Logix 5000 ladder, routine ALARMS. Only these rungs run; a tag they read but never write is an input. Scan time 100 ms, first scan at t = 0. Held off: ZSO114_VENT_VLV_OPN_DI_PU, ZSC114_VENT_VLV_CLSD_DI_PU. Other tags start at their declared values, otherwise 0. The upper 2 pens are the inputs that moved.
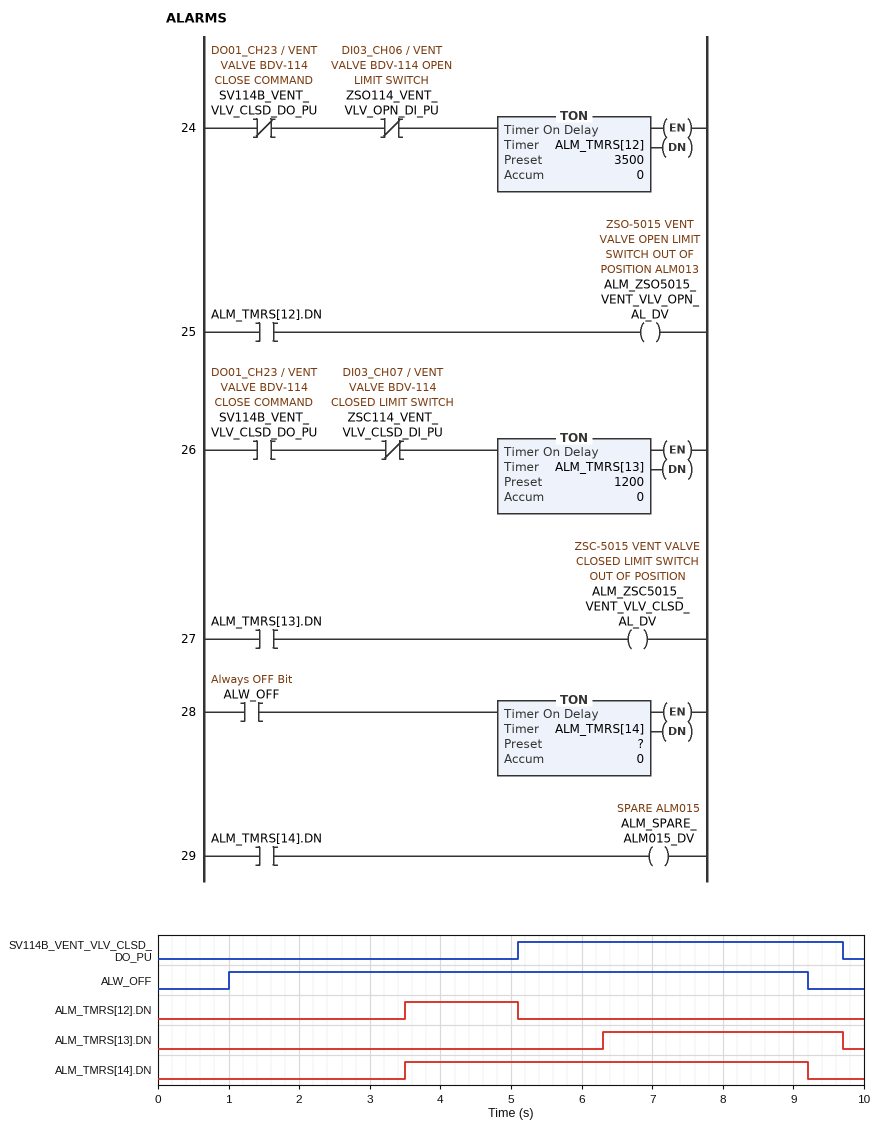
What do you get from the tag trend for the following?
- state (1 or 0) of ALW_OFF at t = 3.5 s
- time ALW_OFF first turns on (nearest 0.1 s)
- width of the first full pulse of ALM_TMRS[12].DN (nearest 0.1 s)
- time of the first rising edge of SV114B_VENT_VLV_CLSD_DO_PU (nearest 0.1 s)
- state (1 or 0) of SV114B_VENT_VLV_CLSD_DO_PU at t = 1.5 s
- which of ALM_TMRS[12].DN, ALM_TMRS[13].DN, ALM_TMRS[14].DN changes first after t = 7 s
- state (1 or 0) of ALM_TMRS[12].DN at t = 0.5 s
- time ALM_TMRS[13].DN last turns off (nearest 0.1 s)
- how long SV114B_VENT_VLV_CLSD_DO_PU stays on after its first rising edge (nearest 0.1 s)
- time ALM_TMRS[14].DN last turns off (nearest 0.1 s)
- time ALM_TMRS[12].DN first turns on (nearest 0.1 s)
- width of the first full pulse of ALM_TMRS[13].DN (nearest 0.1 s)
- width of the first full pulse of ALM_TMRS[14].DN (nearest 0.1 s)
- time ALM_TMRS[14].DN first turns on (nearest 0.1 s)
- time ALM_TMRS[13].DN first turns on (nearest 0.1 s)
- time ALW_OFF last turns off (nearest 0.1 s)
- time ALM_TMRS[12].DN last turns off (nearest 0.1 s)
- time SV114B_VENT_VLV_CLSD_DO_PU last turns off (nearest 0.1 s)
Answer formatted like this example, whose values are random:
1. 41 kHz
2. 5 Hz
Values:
1. 1
2. 1.0 s
3. 1.6 s
4. 5.1 s
5. 0
6. ALM_TMRS[14].DN
7. 0
8. 9.7 s
9. 4.6 s
10. 9.2 s
11. 3.5 s
12. 3.4 s
13. 5.7 s
14. 3.5 s
15. 6.3 s
16. 9.2 s
17. 5.1 s
18. 9.7 s
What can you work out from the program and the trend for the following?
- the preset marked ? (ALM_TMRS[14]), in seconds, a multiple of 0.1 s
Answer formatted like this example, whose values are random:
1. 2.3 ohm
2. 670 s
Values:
1. 2.5 s
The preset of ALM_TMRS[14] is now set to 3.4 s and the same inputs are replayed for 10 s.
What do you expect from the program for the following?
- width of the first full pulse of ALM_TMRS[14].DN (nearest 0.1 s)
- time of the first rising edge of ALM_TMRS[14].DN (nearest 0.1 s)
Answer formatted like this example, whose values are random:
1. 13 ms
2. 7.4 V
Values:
1. 4.8 s
2. 4.4 s
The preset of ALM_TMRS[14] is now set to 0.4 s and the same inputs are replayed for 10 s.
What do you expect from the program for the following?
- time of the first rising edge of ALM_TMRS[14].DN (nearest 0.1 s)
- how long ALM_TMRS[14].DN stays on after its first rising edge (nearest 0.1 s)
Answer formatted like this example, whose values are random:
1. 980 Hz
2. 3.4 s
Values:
1. 1.4 s
2. 7.8 s
